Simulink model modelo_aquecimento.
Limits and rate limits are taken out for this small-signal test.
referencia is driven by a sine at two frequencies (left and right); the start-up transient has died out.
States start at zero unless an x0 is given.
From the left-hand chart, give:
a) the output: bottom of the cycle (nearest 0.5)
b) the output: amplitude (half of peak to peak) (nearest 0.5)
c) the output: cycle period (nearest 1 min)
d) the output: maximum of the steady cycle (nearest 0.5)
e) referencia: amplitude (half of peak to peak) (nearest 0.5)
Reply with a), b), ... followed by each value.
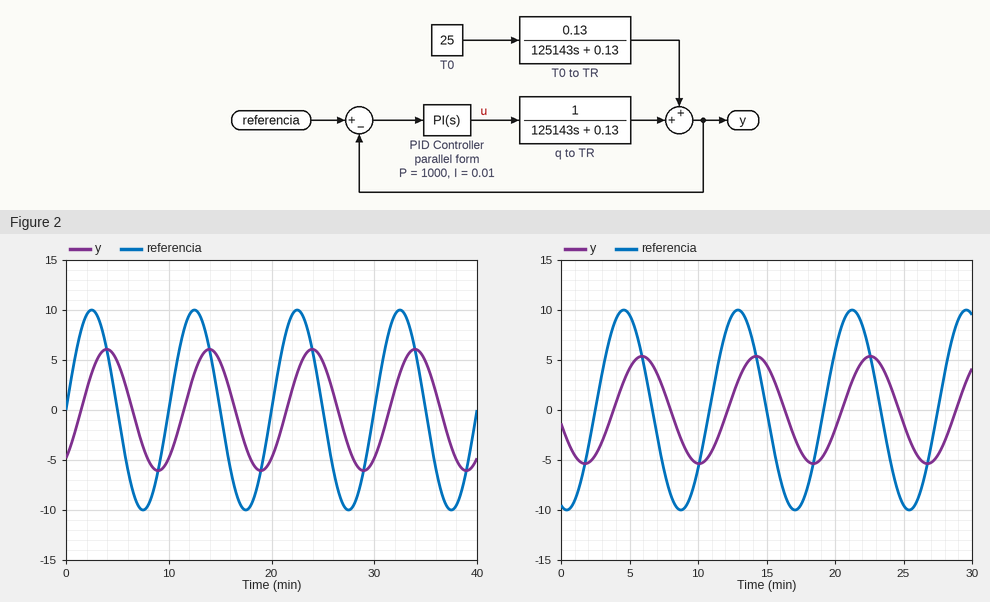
a) -6.0
b) 6.0
c) 10 min
d) 6.0
e) 10.0
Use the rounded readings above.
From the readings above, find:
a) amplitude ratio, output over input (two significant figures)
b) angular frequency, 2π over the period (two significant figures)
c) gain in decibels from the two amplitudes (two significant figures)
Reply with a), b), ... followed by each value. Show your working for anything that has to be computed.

a) 6 / 10 = 0.60
b) 2π / 10 = 0.63 rad/min
c) 20 log10(6 / 10) = -4.4 dB
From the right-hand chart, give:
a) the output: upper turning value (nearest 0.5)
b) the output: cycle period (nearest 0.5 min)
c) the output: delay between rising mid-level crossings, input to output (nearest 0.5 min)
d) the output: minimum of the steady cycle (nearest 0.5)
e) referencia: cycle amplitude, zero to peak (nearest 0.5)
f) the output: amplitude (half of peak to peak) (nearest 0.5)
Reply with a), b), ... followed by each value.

a) 5.5
b) 8.5 min
c) 1.5 min
d) -5.5
e) 10.0
f) 5.5
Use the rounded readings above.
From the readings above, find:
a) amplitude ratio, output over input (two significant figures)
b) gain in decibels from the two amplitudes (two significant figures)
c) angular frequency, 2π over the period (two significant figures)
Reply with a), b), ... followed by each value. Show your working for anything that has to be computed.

a) 5.5 / 10 = 0.55
b) 20 log10(5.5 / 10) = -5.2 dB
c) 2π / 8.5 = 0.74 rad/min
